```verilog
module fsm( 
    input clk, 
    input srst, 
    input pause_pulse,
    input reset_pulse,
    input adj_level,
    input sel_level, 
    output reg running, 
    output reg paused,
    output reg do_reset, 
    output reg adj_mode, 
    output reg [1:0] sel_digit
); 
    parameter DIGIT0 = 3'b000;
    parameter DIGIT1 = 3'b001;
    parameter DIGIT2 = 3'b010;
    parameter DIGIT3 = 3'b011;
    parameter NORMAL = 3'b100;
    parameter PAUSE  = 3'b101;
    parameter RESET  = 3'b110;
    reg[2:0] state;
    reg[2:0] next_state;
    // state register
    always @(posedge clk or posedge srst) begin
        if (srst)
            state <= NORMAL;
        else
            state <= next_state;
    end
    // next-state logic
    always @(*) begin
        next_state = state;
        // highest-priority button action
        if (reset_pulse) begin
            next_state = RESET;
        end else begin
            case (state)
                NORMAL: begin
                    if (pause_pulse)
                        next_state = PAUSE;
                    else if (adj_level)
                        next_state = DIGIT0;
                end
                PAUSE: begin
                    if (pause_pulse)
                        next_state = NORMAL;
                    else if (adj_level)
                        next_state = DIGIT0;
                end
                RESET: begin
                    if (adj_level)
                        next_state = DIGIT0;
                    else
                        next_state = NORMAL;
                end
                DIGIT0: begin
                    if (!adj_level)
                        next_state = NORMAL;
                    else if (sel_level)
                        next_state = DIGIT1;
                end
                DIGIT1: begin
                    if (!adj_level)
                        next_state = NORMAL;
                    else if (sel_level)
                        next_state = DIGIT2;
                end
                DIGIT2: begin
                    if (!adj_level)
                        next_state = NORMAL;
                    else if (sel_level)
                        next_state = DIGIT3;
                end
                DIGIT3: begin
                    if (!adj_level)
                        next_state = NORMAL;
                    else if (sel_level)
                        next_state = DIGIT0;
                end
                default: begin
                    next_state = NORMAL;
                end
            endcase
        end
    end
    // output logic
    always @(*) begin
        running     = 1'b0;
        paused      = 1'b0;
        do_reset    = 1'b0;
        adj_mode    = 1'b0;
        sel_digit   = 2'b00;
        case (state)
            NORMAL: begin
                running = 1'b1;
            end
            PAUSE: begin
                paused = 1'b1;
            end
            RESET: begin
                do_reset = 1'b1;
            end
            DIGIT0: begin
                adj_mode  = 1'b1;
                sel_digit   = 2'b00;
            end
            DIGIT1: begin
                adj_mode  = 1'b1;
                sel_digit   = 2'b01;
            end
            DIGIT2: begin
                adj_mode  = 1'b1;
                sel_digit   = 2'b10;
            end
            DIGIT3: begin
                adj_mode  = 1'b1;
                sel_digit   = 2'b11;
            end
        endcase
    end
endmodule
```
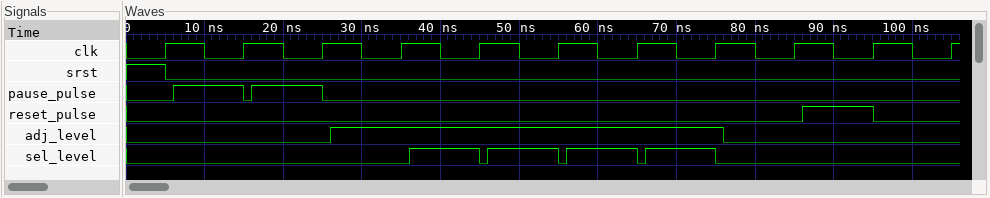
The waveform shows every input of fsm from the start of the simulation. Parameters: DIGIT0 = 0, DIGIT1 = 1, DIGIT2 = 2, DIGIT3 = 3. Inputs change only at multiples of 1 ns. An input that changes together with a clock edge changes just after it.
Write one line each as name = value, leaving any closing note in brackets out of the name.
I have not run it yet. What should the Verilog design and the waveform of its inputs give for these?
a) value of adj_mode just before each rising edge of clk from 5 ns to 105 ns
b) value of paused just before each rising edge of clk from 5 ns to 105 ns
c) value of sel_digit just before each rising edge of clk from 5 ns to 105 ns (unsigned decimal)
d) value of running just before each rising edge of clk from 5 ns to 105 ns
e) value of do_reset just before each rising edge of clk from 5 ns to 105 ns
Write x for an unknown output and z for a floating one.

value of adj_mode just before each rising edge of clk from 5 ns to 105 ns = 0 0 0 0 1 1 1 1 1 0 0
value of paused just before each rising edge of clk from 5 ns to 105 ns = 0 0 1 0 0 0 0 0 0 0 0
value of sel_digit just before each rising edge of clk from 5 ns to 105 ns = 0, 0, 0, 0, 0, 1, 2, 3, 0, 0, 0
value of running just before each rising edge of clk from 5 ns to 105 ns = 1 1 0 1 0 0 0 0 0 1 0
value of do_reset just before each rising edge of clk from 5 ns to 105 ns = 0 0 0 0 0 0 0 0 0 0 1
